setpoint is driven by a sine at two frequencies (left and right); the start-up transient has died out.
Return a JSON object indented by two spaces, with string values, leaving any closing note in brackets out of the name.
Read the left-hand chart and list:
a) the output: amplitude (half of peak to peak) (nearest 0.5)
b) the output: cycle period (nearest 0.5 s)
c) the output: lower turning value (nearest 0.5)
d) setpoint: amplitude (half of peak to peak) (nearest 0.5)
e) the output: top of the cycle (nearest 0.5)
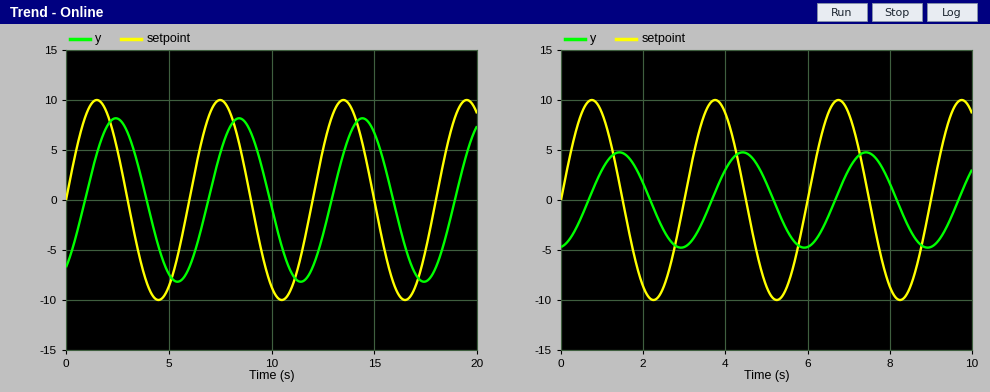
{
  "the output: amplitude (half of peak to peak)": "8.0",
  "the output: cycle period": "6.0 s",
  "the output: lower turning value": "-8.0",
  "setpoint: amplitude (half of peak to peak)": "10.0",
  "the output: top of the cycle": "8.0"
}
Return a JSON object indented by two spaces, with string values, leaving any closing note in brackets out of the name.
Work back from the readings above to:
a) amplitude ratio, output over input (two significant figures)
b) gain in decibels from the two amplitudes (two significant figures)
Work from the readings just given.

{
  "amplitude ratio, output over input": "0.80",
  "gain in decibels from the two amplitudes": "-1.9 dB"
}
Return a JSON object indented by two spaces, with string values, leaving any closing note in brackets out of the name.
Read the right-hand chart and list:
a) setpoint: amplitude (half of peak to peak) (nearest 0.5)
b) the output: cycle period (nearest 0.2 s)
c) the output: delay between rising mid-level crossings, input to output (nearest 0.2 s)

{
  "setpoint: amplitude (half of peak to peak)": "10.0",
  "the output: cycle period": "3.0 s",
  "the output: delay between rising mid-level crossings, input to output": "0.6 s"
}
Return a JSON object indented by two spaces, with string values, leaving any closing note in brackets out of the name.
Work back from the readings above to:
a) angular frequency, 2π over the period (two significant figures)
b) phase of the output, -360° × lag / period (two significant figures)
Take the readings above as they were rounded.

{
  "angular frequency, 2π over the period": "2.1 rad/s",
  "phase of the output, -360° × lag / period": "-72°"
}
